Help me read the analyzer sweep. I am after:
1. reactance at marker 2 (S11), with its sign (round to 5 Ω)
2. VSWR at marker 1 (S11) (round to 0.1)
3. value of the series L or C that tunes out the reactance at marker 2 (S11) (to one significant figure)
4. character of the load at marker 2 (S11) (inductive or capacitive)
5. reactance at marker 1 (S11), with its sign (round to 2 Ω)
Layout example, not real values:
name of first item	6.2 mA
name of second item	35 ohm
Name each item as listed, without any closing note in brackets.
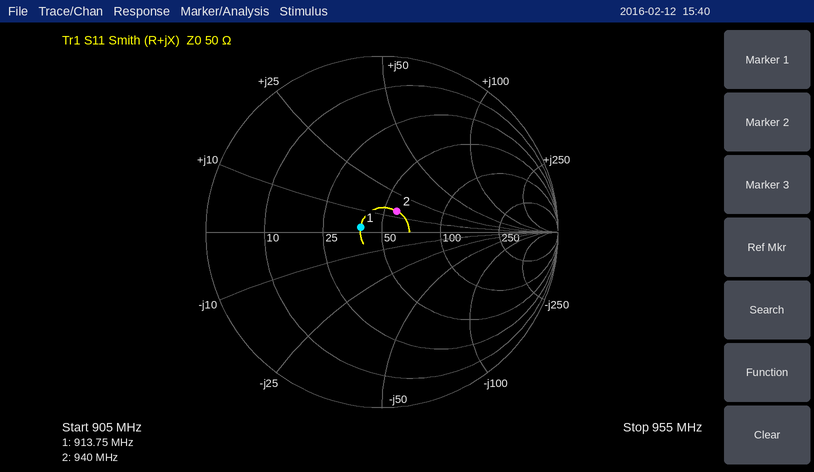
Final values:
reactance at marker 2 (S11), with its sign	+15 Ω
VSWR at marker 1 (S11)	1.3
value of the series L or C that tunes out the reactance at marker 2 (S11)	10 pF
character of the load at marker 2 (S11)	inductive
reactance at marker 1 (S11), with its sign	+2 Ω
